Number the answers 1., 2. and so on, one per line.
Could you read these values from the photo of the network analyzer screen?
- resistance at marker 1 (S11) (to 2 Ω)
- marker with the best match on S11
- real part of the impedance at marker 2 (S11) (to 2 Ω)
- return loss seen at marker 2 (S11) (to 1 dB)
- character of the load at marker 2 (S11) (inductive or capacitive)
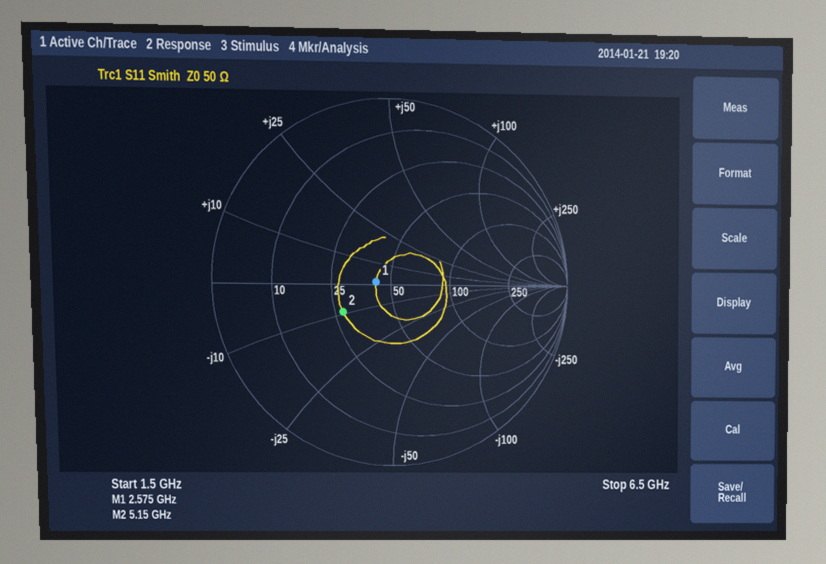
1. 42 Ω
2. marker 1
3. 28 Ω
4. 10 dB
5. capacitive
